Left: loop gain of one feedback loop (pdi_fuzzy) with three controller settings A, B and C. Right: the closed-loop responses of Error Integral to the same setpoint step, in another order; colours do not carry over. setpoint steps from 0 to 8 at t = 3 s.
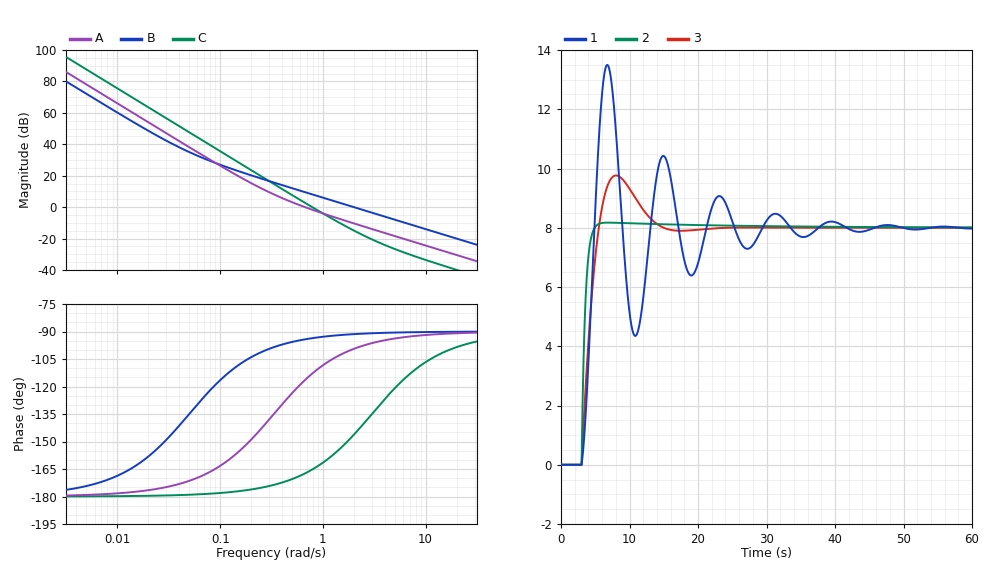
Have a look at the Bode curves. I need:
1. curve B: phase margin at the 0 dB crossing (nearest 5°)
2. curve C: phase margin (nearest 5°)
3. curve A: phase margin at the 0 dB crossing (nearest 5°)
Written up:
90°
15°
65°
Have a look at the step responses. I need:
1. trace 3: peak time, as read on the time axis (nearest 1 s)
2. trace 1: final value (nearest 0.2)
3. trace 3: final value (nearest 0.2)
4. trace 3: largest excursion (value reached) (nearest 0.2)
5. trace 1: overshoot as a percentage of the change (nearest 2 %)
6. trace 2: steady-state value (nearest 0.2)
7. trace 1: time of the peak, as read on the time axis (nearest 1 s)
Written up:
8 s
8.0
8.0
9.8
68 %
8.0
7 s
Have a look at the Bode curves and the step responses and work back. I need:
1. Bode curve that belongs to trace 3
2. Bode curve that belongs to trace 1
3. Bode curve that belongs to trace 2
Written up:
A
C
B
